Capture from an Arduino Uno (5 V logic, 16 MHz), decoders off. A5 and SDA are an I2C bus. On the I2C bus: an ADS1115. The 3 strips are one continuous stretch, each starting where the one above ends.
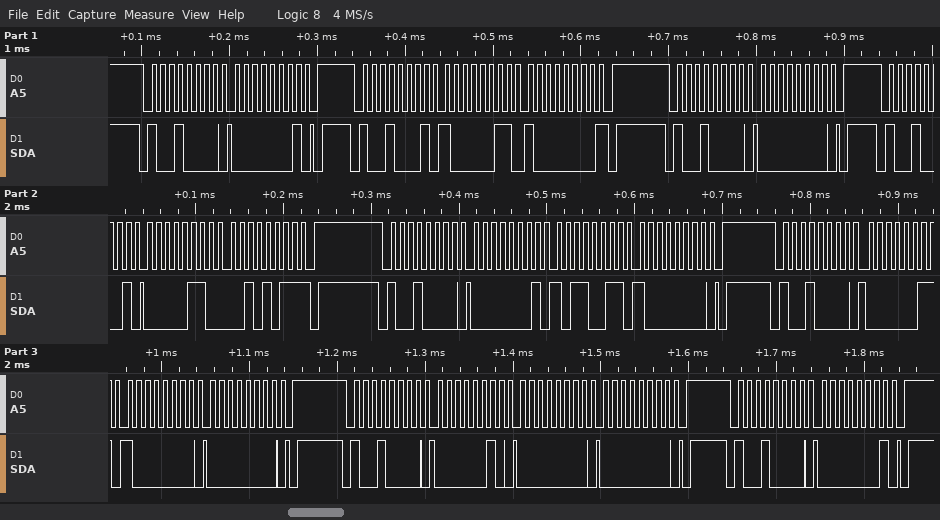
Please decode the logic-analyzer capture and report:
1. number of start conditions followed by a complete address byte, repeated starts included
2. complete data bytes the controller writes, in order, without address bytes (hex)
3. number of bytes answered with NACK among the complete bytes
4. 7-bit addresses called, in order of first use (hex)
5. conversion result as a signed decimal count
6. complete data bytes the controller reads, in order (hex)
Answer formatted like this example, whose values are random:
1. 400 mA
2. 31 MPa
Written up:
1. 8
2. 01 00 01 B3 80 03 80 00 02 00 00 01
3. 2
4. 0x48
5. 1579
6. 83 80 06 2B
